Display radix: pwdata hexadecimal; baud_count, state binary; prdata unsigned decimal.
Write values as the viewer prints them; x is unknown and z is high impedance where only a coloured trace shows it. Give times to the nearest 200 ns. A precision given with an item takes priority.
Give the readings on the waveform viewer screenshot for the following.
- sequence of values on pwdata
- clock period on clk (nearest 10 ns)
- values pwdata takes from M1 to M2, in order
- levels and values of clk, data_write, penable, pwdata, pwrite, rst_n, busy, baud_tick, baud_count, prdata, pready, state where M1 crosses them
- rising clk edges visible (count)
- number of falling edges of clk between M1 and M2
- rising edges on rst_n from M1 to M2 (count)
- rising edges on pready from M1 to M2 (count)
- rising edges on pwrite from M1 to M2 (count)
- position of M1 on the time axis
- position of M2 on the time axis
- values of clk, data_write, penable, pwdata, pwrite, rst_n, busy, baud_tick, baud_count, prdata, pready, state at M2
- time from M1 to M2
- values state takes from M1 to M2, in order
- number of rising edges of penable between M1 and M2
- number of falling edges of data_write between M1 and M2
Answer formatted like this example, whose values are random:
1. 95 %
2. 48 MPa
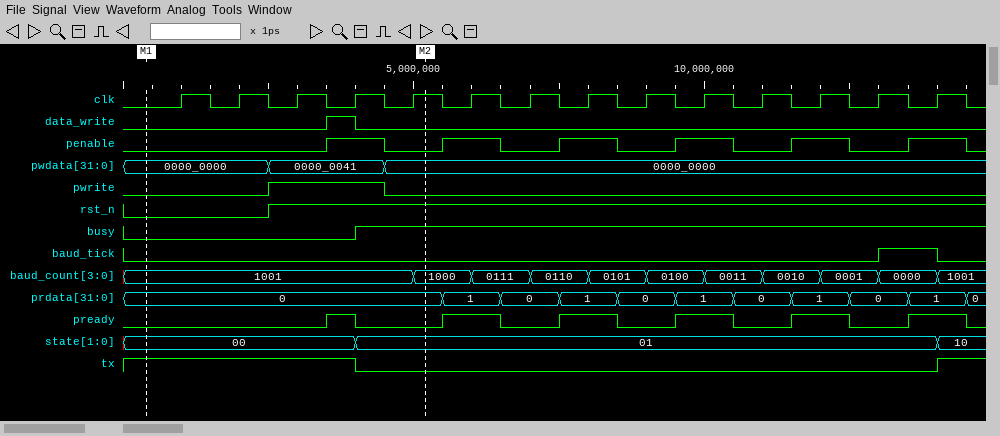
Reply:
1. 0000_0000, 0000_0041, 0000_0000
2. 1000 ns
3. 0000_0000, 0000_0041, 0000_0000
4. clk=0, data_write=0, penable=0, pwdata=0000_0000, pwrite=0, rst_n=0, busy=0, baud_tick=0, baud_count=1001, prdata=0, pready=0, state=00
5. 14
6. 4
7. 1
8. 1
9. 1
10. 400 ns
11. 5200 ns
12. clk=1, data_write=0, penable=0, pwdata=0000_0000, pwrite=0, rst_n=1, busy=1, baud_tick=0, baud_count=1000, prdata=0, pready=0, state=01
13. 4800 ns
14. 00, 01
15. 1
16. 1
